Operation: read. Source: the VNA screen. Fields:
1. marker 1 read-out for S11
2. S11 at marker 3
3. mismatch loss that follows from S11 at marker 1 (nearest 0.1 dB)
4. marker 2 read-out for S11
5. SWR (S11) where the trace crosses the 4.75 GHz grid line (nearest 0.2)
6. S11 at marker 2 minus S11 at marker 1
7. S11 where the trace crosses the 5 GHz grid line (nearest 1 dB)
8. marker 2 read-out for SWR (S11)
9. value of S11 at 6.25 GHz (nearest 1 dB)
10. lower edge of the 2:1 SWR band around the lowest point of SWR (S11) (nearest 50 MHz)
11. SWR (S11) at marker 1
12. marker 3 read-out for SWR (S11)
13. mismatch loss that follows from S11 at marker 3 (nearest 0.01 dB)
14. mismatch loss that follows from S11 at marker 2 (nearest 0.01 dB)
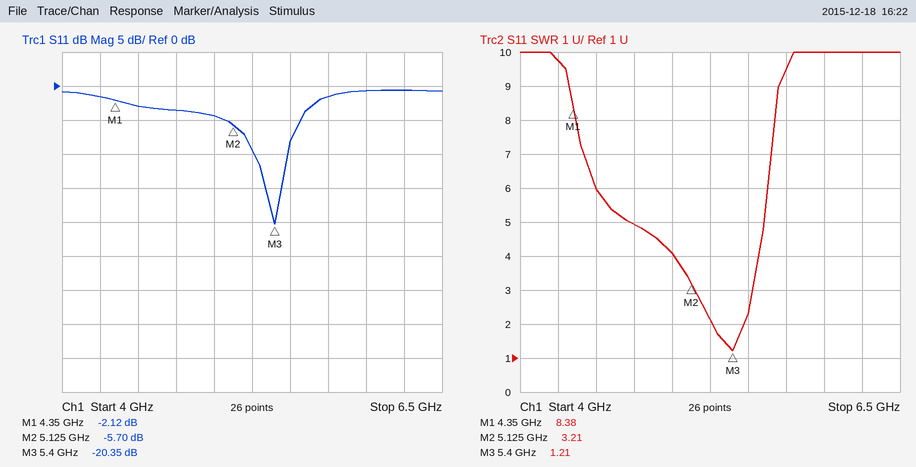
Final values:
-2.12 dB
-20.35 dB
4.1 dB
-5.70 dB
5.0
-3.58 dB
-4 dB
3.21
-1 dB
5.25 GHz
8.38
1.21
0.04 dB
1.36 dB
